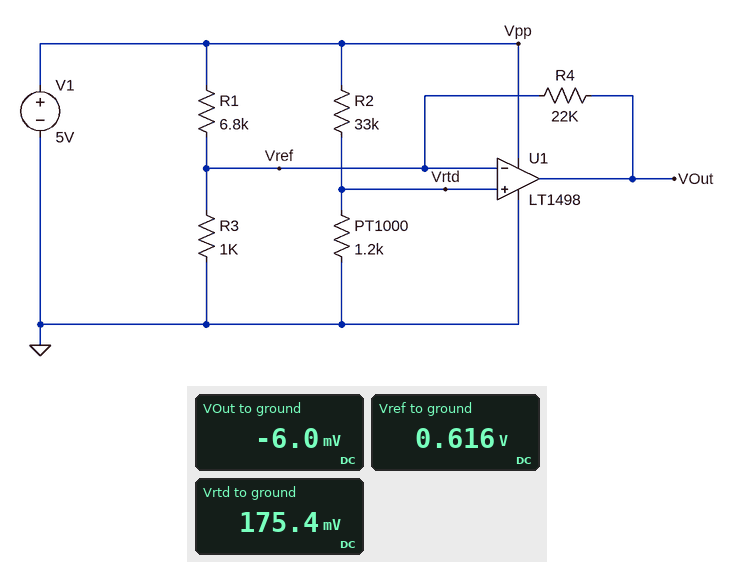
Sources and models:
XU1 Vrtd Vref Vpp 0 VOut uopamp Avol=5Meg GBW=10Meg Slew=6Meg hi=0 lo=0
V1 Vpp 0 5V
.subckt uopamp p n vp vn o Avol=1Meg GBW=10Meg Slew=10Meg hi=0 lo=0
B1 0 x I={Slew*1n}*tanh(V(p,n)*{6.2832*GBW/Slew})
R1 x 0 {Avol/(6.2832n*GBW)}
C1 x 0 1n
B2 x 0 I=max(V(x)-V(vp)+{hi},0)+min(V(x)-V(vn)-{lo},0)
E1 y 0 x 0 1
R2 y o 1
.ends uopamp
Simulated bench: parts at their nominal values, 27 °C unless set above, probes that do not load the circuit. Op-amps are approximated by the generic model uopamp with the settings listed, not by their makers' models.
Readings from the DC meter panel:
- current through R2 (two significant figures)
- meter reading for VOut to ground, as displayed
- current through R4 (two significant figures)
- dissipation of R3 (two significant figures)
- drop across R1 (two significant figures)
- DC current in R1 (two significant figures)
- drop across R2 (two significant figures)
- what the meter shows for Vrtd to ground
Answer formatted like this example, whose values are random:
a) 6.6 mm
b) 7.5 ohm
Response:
a) 150 µA
b) -6.0 mV
c) 28 µA
d) 380 µW
e) 4.4 V
f) 640 µA
g) 4.8 V
h) 175.4 mV
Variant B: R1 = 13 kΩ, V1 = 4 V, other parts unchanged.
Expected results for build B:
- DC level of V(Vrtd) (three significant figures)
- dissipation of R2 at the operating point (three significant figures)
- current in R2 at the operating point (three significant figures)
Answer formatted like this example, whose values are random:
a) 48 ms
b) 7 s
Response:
a) 140 mV
b) 451 µW
c) 117 µA
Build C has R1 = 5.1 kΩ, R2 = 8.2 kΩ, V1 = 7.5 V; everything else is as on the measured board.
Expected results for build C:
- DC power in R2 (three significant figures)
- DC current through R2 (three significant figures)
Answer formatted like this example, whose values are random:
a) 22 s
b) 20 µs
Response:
a) 5.22 mW
b) 798 µA
